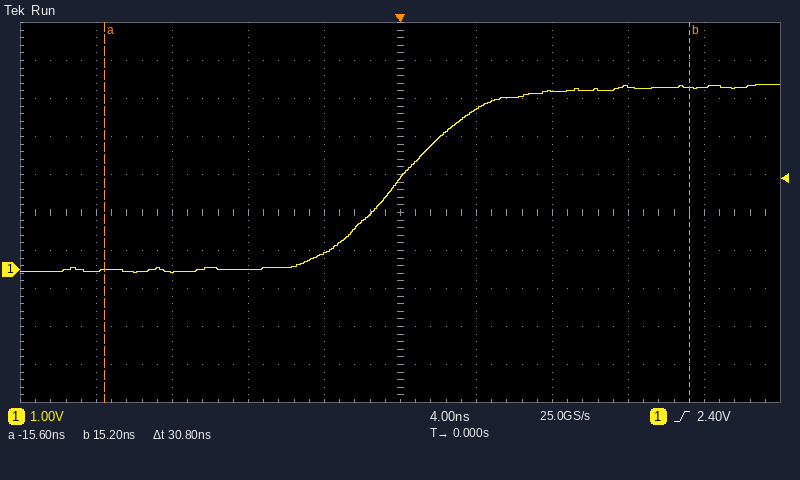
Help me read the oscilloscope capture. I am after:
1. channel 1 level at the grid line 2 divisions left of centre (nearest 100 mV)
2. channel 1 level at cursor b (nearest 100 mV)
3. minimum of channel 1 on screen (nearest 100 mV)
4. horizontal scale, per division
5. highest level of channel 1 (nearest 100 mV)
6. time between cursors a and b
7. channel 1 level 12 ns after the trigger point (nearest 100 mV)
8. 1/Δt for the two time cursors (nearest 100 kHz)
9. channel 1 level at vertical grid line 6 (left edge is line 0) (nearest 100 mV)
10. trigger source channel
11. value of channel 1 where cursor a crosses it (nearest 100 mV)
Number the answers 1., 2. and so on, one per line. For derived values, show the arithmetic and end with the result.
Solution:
1. 0.0 V
2. 4.8 V
3. -100 mV
4. 4 ns
5. 4.9 V
6. 30.8 ns
7. 4.8 V
8. 1 / 30.8 ns ≈ 32.5 MHz
9. 4.2 V
10. channel 1
11. 0.0 V
